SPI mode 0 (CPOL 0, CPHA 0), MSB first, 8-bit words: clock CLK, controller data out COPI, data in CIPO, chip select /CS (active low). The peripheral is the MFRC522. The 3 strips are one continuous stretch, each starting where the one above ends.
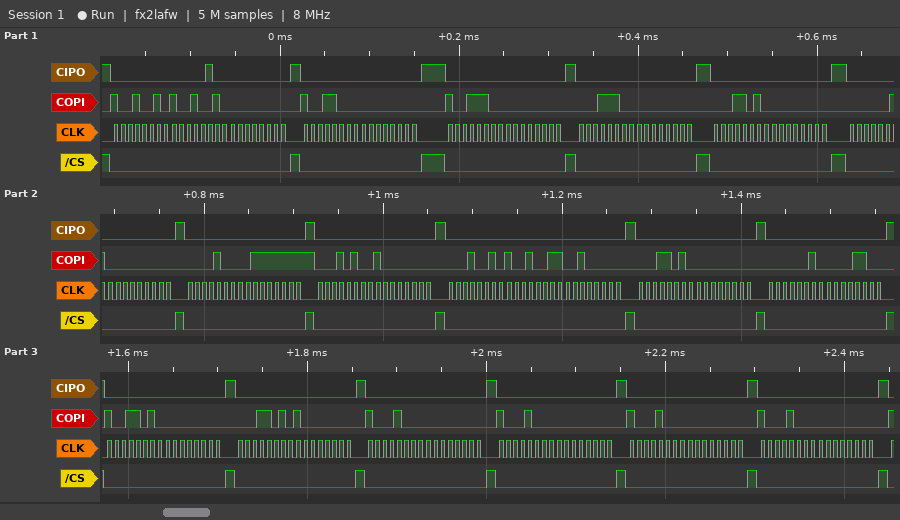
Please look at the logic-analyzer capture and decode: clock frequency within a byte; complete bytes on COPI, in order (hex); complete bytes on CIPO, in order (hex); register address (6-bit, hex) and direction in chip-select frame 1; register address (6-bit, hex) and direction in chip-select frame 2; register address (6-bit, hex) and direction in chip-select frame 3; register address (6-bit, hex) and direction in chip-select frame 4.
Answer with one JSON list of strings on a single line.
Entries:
["125 kHz", "0x92 0x92 0x00 0x98 0x00 0x9C 0x00 0x1C 0x00 0x1A 0x00 0x02 0x00 0x08 0x7F 0x14 0x80 0x12 0x93 0x20 0x1A 0x00 0x02 0x0C 0x9A 0x00 0x1A 0x80 0x88 0x00 0x88 0x00 0x88 0x00 0x88 0x00", "0x00 0x04 0x00 0x00 0x00 0x00 0x00 0x00 0x00 0x00 0x00 0x00 0x00 0x00 0x00 0x00 0x00 0x00 0x00 0x00 0x00 0x00 0x00 0x00 0x00 0x00 0x00 0x00 0x00 0x00 0x00 0x00 0x00 0x00 0x00 0x00", "0x09 read", "0x0C read", "0x0E read", "0x0E write"]
